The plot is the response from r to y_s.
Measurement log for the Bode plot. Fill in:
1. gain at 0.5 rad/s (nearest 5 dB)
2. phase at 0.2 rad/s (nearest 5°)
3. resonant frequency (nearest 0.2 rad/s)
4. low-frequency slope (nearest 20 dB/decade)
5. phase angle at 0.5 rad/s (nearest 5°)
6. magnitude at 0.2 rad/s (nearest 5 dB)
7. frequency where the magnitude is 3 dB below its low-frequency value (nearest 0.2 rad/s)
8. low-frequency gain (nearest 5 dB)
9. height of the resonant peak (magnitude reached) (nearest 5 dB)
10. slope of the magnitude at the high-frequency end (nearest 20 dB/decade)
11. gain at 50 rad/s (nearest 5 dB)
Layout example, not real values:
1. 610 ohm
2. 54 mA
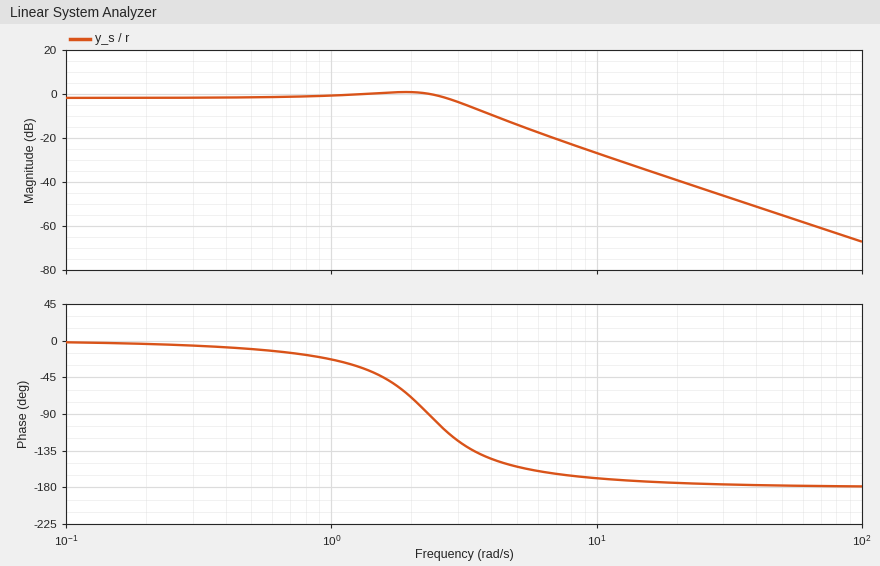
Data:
1. 0 dB
2. -5°
3. 1.8 rad/s
4. 0 dB/decade
5. -10°
6. 0 dB
7. 3.2 rad/s
8. 0 dB
9. 0 dB
10. -40 dB/decade
11. -55 dB
